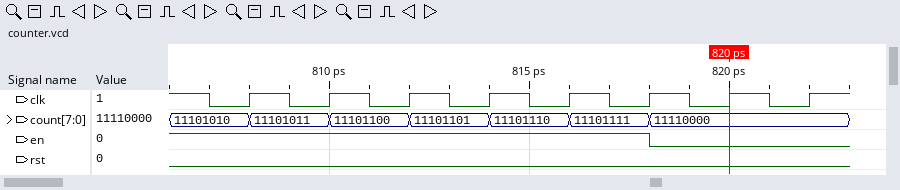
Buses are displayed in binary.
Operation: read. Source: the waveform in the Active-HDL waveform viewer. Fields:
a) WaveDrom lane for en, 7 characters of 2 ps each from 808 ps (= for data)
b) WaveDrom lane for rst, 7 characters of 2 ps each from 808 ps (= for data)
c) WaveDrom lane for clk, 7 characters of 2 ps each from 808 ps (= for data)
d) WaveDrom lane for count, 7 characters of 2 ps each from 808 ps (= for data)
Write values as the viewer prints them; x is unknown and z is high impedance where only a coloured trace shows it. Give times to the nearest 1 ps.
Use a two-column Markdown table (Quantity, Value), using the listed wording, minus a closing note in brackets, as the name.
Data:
| Quantity | Value |
|---|---|
| WaveDrom lane for en, 7 characters of 2 ps each from 808 ps | {name: 'en', wave: '1....0.'} |
| WaveDrom lane for rst, 7 characters of 2 ps each from 808 ps | {name: 'rst', wave: '0......'} |
| WaveDrom lane for clk, 7 characters of 2 ps each from 808 ps | {name: 'clk', wave: 'p......'} |
| WaveDrom lane for count, 7 characters of 2 ps each from 808 ps | {name: 'count', wave: '======.', data: '11101011 11101100 11101101 11101110 11101111 11110000'} |
